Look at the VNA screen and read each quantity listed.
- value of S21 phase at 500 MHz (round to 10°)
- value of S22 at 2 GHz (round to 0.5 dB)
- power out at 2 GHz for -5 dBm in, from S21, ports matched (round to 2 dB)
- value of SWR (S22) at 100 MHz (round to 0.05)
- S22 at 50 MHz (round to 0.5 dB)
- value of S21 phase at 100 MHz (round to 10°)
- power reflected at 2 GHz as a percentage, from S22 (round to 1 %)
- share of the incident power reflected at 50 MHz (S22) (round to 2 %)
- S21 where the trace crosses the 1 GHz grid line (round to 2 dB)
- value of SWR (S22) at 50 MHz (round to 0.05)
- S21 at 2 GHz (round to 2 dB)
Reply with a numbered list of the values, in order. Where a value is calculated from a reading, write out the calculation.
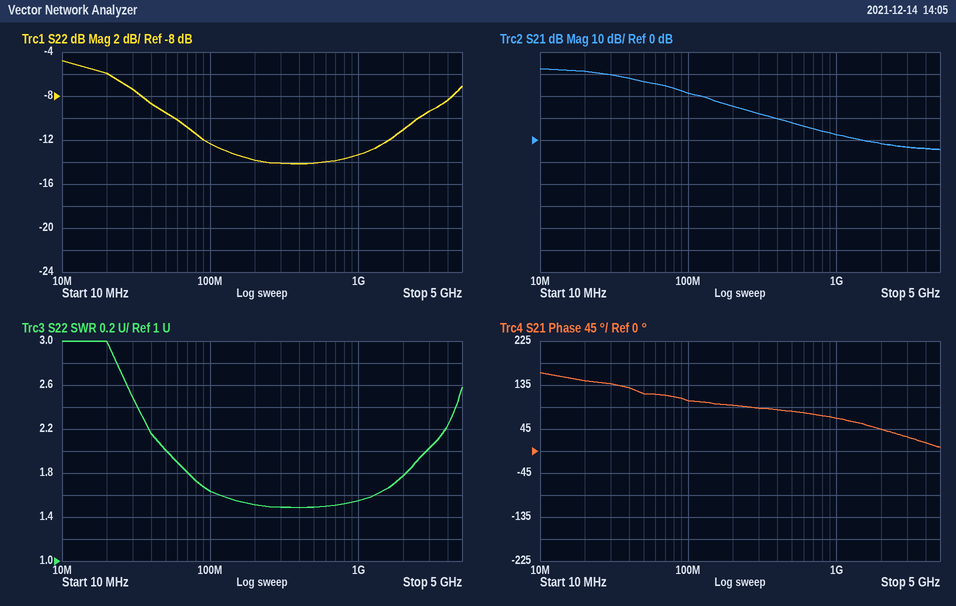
1. 80°
2. -11.0 dB
3. -5 dBm + (-2 dB) = -6 dBm
4. 1.65
5. -9.5 dB
6. 100°
7. 10^(-11/10) ≈ 8 %
8. 10^(-9.5/10) ≈ 11.2 %, so 12 % to the nearest 2 %
9. 2 dB
10. 2.00
11. -2 dB
